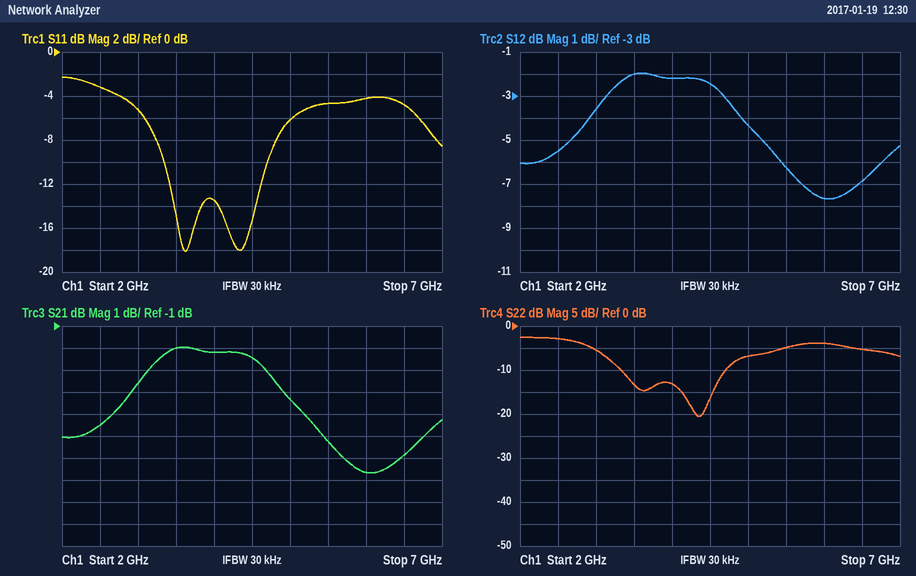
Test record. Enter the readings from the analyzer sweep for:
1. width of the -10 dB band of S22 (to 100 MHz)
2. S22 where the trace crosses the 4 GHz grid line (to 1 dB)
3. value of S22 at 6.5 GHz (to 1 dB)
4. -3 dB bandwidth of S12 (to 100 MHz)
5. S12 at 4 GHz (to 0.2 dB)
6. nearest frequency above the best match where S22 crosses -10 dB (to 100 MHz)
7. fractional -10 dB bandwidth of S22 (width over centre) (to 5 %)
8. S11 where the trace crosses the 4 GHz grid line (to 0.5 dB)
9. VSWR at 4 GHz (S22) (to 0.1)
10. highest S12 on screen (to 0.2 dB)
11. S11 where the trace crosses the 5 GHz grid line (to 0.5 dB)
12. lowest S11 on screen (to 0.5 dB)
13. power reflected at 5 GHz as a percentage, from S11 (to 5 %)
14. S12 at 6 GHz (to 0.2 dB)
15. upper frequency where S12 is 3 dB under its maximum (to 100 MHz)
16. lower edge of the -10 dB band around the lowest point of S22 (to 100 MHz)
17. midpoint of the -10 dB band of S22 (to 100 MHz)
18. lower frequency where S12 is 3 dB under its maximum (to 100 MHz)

1.4 GHz
-13 dB
-5 dB
2.5 GHz
-2.2 dB
4.7 GHz
35 %
-13.5 dB
1.6
-2.0 dB
-6.0 dB
-18.0 dB
25 %
-7.6 dB
5.2 GHz
3.3 GHz
4.0 GHz
2.7 GHz
